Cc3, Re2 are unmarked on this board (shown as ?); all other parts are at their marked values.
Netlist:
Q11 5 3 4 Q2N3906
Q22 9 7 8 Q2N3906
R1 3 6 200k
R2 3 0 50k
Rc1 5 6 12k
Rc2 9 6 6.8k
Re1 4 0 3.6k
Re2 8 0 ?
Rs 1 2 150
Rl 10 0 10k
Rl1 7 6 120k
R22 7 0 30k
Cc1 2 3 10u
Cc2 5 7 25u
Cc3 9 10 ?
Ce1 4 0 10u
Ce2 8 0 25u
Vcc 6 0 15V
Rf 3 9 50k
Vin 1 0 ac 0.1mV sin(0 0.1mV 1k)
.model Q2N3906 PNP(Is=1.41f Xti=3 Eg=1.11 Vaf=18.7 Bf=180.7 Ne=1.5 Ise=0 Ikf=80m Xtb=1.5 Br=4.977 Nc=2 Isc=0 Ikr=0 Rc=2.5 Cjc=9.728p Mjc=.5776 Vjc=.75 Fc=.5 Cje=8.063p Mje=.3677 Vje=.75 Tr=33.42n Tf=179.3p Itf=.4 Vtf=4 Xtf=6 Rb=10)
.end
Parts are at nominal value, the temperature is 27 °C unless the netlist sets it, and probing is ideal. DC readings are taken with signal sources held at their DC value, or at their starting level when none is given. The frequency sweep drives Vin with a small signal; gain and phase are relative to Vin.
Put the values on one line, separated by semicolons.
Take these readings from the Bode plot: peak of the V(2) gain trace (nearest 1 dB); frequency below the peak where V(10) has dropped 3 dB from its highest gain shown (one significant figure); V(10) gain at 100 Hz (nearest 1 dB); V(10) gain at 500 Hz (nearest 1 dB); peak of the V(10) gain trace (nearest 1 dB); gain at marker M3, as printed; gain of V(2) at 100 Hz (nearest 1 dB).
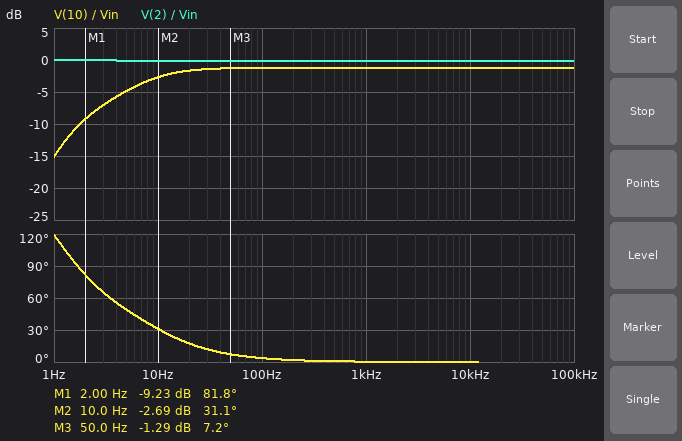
0 dB; 6 Hz; -1 dB; -1 dB; -1 dB; -1.29 dB; 0 dB
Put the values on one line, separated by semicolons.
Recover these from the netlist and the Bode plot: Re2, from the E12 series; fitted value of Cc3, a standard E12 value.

10 kΩ; 22 µF
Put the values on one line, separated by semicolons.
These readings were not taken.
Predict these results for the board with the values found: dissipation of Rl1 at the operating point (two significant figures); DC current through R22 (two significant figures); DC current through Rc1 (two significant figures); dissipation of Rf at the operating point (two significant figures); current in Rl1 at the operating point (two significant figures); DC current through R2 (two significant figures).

480 µW; 250 µA; 570 µA; 9.2 µW; 63 µA; 150 µA
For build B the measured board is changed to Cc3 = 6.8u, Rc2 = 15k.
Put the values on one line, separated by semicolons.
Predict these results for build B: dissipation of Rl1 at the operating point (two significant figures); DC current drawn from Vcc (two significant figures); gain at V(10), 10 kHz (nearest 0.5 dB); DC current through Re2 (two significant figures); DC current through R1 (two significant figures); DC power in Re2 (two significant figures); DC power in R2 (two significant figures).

750 µW; 1.3 mA; 0 dB; 500 µA; 41 µA; 2.5 mW; 930 µW
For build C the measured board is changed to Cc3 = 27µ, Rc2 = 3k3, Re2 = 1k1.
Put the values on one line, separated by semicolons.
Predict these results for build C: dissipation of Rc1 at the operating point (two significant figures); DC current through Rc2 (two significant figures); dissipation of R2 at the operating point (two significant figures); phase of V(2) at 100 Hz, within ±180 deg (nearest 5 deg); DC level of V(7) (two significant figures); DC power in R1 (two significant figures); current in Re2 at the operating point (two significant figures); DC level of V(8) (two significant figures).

3.2 mW; 1.5 mA; 1.3 mW; 0 deg; 9.2 V; 240 µW; 1.2 mA; 1.4 V
